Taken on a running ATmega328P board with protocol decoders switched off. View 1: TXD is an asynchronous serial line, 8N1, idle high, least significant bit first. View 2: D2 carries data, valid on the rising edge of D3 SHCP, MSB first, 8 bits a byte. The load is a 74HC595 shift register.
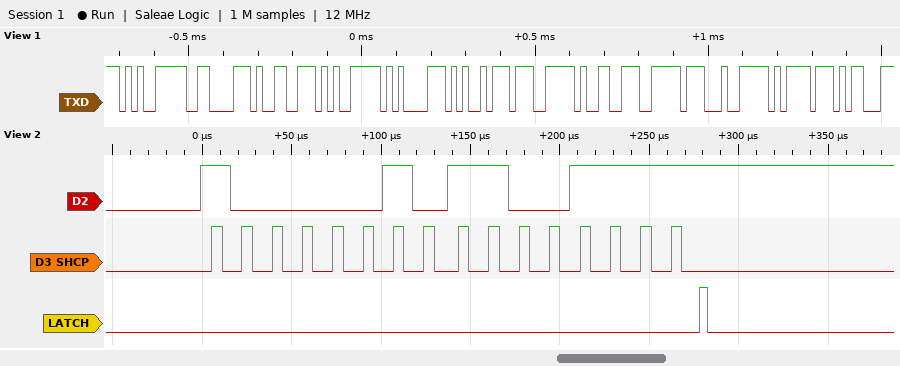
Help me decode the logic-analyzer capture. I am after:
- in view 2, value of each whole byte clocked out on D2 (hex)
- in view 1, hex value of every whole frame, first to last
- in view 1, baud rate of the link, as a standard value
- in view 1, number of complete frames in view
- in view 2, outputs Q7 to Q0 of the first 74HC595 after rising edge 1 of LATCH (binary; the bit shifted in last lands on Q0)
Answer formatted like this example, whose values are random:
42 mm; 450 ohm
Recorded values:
82 CF; E5 86 99 E5 85 A5 E7 99 BE E4 BD 8D; 57600 baud; 12; 11001111
